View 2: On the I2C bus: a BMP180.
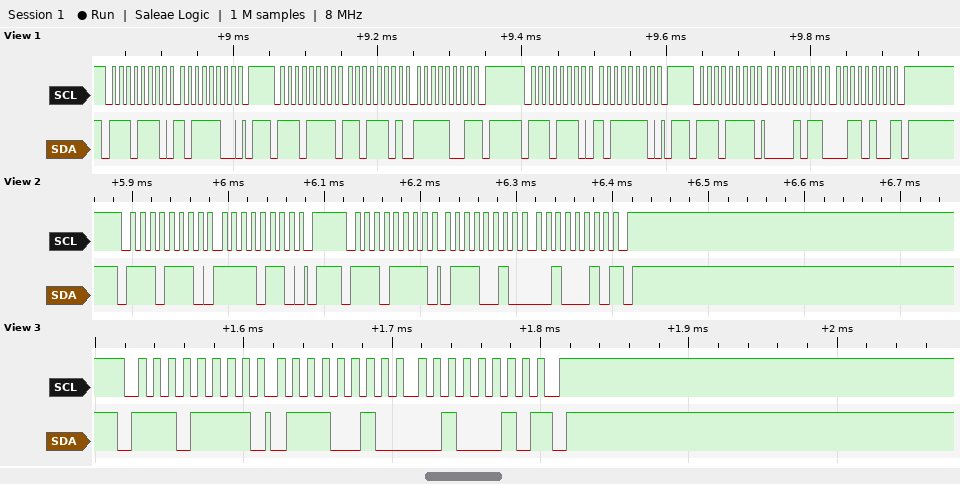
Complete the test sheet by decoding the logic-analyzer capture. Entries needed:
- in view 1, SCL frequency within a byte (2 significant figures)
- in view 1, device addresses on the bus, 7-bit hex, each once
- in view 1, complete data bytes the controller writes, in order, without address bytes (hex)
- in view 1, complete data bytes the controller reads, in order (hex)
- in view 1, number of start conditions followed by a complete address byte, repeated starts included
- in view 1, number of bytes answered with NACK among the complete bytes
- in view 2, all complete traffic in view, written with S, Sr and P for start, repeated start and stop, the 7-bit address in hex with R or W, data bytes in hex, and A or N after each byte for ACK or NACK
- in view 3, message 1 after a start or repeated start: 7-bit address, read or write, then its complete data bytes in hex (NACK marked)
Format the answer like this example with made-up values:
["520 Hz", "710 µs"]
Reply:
["100 kHz", "0x77", "BC BE", "DD F9 0B 34", "4", "2", "S 77W A F6 A P S 77R A 72 A 22 N P", "0x77 read: 72 22 NACK"]
